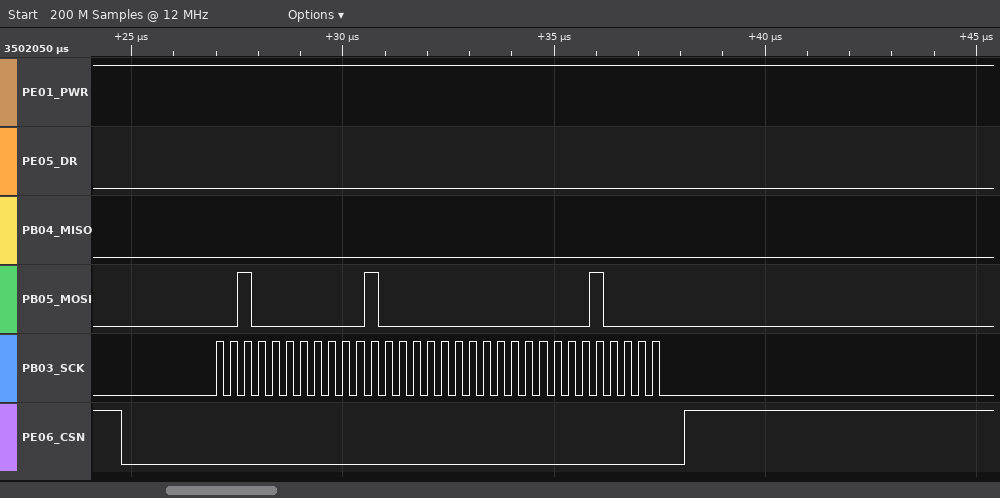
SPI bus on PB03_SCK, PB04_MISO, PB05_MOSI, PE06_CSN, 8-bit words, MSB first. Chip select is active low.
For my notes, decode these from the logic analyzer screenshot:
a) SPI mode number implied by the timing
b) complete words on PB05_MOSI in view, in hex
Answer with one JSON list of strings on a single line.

["0", "20, 10, 00, 10"]
